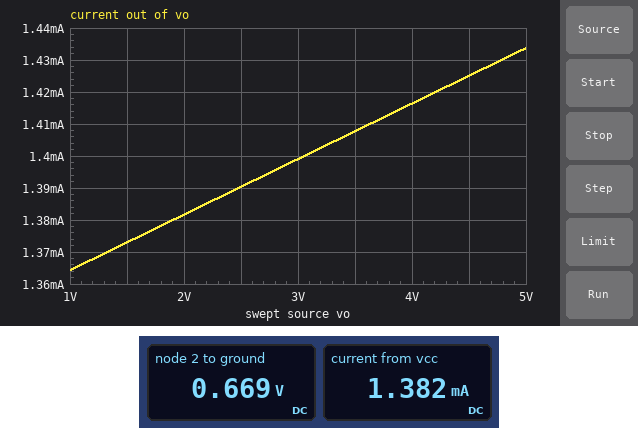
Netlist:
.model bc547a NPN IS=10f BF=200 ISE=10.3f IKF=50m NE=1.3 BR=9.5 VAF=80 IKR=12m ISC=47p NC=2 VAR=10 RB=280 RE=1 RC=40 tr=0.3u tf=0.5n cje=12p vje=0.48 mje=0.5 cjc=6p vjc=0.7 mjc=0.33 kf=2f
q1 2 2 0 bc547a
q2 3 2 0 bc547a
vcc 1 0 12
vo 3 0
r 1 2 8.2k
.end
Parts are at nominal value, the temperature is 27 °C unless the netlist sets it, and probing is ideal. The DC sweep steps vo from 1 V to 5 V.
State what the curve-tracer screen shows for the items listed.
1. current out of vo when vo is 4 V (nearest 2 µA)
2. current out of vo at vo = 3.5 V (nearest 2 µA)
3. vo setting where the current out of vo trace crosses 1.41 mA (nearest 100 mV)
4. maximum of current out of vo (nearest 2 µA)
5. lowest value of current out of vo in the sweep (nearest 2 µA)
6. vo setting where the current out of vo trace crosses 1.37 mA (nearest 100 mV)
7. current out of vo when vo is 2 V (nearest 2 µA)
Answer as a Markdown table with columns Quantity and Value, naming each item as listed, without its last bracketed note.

| Quantity | Value |
|---|---|
| current out of vo when vo is 4 V | 1.416 mA |
| current out of vo at vo = 3.5 V | 1.408 mA |
| vo setting where the current out of vo trace crosses 1.41 mA | 3.6 V |
| maximum of current out of vo | 1.434 mA |
| lowest value of current out of vo in the sweep | 1.364 mA |
| vo setting where the current out of vo trace crosses 1.37 mA | 1.3 V |
| current out of vo when vo is 2 V | 1.382 mA |
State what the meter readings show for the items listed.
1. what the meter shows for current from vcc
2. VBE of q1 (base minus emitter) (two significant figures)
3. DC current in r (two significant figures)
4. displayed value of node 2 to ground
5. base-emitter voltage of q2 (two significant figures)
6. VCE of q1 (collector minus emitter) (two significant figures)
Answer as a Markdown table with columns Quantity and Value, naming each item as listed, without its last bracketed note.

| Quantity | Value |
|---|---|
| what the meter shows for current from vcc | 1.382 mA |
| VBE of q1 (base minus emitter) | 670 mV |
| DC current in r | 1.4 mA |
| displayed value of node 2 to ground | 0.669 V |
| base-emitter voltage of q2 | 670 mV |
| VCE of q1 (collector minus emitter) | 670 mV |
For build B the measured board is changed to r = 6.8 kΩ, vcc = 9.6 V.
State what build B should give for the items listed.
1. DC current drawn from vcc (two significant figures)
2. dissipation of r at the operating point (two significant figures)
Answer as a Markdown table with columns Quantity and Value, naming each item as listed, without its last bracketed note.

| Quantity | Value |
|---|---|
| DC current drawn from vcc | 1.3 mA |
| dissipation of r at the operating point | 12 mW |
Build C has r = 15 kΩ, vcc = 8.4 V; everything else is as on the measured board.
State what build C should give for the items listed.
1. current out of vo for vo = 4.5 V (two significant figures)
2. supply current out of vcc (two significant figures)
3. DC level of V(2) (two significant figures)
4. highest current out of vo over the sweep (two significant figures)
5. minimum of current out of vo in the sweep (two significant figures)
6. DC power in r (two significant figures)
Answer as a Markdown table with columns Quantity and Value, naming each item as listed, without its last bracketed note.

| Quantity | Value |
|---|---|
| current out of vo for vo = 4.5 V | 530 µA |
| supply current out of vcc | 520 µA |
| DC level of V(2) | 640 mV |
| highest current out of vo over the sweep | 540 µA |
| minimum of current out of vo in the sweep | 510 µA |
| DC power in r | 4.0 mW |
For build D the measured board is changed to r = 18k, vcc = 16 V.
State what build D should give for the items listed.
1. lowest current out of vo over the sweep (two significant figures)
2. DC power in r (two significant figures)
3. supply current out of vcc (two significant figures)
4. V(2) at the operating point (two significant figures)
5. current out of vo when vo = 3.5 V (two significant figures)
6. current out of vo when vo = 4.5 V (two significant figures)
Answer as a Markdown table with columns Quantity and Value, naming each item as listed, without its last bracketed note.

| Quantity | Value |
|---|---|
| lowest current out of vo over the sweep | 840 µA |
| DC power in r | 13 mW |
| supply current out of vcc | 850 µA |
| V(2) at the operating point | 650 mV |
| current out of vo when vo = 3.5 V | 870 µA |
| current out of vo when vo = 4.5 V | 880 µA |
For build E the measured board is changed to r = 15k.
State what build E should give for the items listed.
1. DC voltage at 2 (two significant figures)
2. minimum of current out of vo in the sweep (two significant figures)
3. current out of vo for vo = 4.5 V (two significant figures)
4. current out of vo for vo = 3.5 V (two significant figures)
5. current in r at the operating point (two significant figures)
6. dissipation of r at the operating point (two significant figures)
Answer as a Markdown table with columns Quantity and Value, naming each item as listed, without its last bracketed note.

| Quantity | Value |
|---|---|
| DC voltage at 2 | 650 mV |
| minimum of current out of vo in the sweep | 750 µA |
| current out of vo for vo = 4.5 V | 780 µA |
| current out of vo for vo = 3.5 V | 770 µA |
| current in r at the operating point | 760 µA |
| dissipation of r at the operating point | 8.6 mW |
